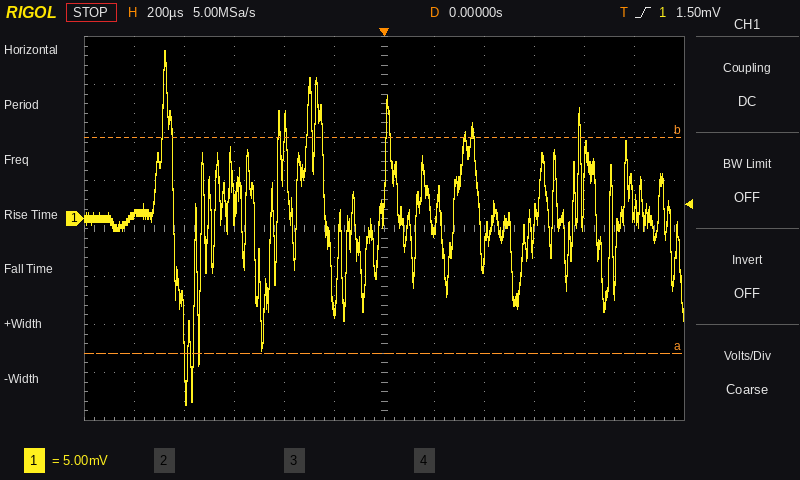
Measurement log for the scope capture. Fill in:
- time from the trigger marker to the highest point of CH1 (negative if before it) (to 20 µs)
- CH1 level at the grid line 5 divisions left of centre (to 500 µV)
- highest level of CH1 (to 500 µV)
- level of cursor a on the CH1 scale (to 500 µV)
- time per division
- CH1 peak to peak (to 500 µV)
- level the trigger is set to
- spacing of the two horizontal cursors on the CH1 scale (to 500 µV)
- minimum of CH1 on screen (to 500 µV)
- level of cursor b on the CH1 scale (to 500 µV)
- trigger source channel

-880 µs
500 µV
17.5 mV
-14.0 mV
200 µs
37.0 mV
1.50 mV
22.5 mV
-19.5 mV
8.5 mV
CH1
